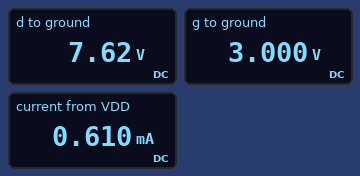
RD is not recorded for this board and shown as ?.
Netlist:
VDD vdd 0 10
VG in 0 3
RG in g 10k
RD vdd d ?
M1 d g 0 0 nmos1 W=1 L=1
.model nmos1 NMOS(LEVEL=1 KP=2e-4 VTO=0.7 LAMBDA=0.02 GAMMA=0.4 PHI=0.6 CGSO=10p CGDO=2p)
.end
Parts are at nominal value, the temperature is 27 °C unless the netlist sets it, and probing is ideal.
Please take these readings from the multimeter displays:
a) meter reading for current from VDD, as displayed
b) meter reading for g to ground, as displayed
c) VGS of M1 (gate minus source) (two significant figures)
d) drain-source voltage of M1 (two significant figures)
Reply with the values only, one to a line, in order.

0.610 mA
3.000 V
3.0 V
7.6 V
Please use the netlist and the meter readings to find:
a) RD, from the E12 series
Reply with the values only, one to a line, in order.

3.9 kΩ
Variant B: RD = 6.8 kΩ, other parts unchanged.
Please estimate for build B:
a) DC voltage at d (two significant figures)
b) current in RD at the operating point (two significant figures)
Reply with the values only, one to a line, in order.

6.0 V
590 µA
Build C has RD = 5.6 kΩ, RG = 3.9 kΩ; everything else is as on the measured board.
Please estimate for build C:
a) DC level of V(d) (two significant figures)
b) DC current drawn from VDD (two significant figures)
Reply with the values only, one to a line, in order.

6.6 V
600 µA
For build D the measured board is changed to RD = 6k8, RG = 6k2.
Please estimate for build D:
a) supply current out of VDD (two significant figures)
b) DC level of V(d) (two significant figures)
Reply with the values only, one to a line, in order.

590 µA
6.0 V
